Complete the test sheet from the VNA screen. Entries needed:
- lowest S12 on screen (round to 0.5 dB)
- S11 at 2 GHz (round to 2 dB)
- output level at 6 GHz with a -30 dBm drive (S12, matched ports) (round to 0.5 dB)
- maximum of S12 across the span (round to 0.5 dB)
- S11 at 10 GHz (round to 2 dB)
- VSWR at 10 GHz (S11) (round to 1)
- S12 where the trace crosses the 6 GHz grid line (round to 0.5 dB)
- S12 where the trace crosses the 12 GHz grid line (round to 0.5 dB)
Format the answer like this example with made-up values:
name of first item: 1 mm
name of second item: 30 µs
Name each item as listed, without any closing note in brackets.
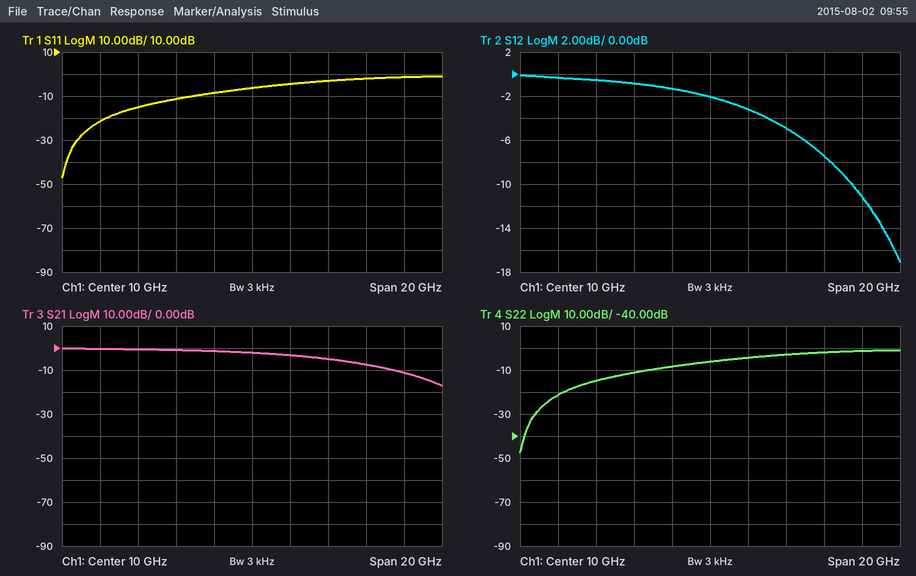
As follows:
lowest S12 on screen: -17.0 dB
S11 at 2 GHz: -22 dB
output level at 6 GHz with a -30 dBm drive (S12, matched ports): -31.0 dBm
maximum of S12 across the span: 0.0 dB
S11 at 10 GHz: -6 dB
VSWR at 10 GHz (S11): 3
S12 where the trace crosses the 6 GHz grid line: -1.0 dB
S12 where the trace crosses the 12 GHz grid line: -3.0 dB
